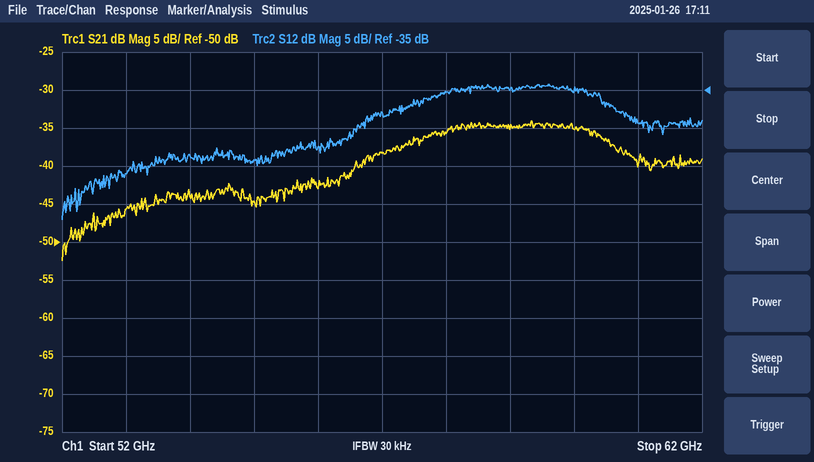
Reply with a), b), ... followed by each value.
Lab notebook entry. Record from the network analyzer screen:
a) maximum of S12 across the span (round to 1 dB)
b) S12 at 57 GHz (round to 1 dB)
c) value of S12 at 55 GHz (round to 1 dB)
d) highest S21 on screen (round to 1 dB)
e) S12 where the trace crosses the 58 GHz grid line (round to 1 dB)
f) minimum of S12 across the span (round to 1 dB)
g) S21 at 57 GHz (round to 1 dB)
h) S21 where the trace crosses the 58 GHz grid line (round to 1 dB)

a) -34 dB
b) -38 dB
c) -44 dB
d) -34 dB
e) -35 dB
f) -52 dB
g) -38 dB
h) -36 dB
